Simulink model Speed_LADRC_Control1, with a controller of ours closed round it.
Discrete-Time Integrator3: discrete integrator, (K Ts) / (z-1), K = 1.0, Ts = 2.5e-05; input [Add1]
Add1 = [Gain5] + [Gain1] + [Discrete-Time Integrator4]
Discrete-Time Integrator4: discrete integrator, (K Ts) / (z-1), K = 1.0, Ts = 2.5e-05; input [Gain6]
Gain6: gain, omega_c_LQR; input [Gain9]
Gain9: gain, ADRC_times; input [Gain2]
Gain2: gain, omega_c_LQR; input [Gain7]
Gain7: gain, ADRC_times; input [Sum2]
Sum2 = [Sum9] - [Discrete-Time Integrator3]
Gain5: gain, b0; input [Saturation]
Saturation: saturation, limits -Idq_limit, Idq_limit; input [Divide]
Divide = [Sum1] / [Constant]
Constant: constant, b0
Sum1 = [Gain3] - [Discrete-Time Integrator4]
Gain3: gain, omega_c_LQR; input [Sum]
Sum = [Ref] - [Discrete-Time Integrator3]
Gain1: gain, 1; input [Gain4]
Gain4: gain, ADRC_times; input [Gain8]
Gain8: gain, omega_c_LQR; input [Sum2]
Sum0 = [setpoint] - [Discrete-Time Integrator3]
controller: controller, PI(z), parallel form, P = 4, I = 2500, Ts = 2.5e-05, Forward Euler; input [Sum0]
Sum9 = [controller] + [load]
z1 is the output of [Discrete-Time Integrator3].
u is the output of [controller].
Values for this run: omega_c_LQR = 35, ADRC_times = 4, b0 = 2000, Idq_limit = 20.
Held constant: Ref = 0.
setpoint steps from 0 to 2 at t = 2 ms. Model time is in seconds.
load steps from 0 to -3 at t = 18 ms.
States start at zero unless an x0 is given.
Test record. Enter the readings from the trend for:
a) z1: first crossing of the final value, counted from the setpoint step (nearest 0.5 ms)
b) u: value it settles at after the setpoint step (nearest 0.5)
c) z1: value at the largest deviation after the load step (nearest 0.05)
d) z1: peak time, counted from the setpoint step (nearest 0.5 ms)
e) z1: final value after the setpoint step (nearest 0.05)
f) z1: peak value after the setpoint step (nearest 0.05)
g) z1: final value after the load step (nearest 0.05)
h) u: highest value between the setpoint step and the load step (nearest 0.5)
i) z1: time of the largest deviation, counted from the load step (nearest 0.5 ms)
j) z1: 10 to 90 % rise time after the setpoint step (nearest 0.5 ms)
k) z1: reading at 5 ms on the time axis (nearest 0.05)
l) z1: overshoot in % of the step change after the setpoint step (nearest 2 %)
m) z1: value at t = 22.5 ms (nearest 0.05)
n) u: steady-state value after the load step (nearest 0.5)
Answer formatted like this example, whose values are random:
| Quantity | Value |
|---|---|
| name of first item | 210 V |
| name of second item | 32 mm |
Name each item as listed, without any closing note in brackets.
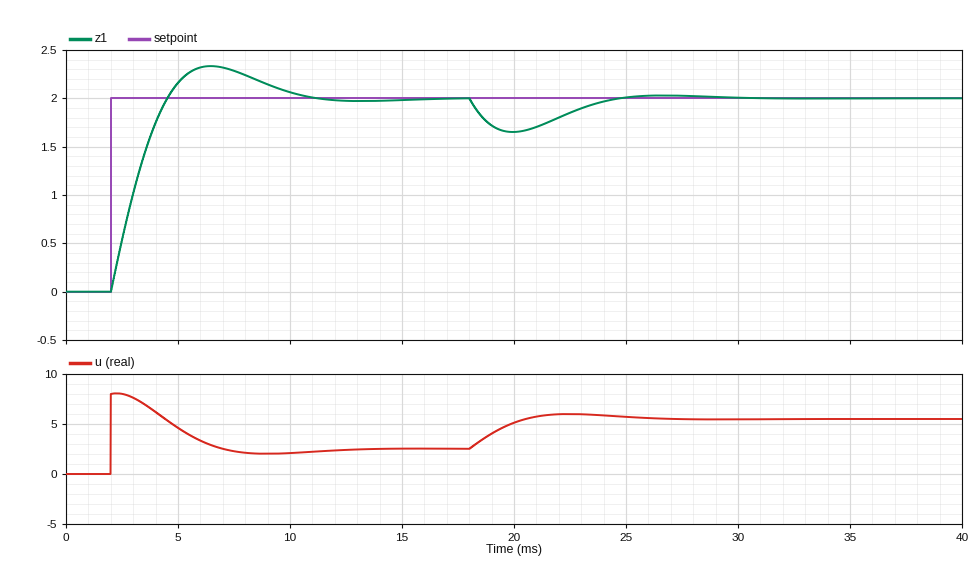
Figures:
| Quantity | Value |
|---|---|
| z1: first crossing of the final value, counted from the setpoint step | 2.5 ms |
| u: value it settles at after the setpoint step | 2.5 |
| z1: value at the largest deviation after the load step | 1.65 |
| z1: peak time, counted from the setpoint step | 4.5 ms |
| z1: final value after the setpoint step | 2.00 |
| z1: peak value after the setpoint step | 2.35 |
| z1: final value after the load step | 2.00 |
| u: highest value between the setpoint step and the load step | 8.0 |
| z1: time of the largest deviation, counted from the load step | 2.0 ms |
| z1: 10 to 90 % rise time after the setpoint step | 2.0 ms |
| z1: reading at 5 ms on the time axis | 2.15 |
| z1: overshoot in % of the step change after the setpoint step | 16 % |
| z1: value at t = 22.5 ms | 1.85 |
| u: steady-state value after the load step | 5.5 |
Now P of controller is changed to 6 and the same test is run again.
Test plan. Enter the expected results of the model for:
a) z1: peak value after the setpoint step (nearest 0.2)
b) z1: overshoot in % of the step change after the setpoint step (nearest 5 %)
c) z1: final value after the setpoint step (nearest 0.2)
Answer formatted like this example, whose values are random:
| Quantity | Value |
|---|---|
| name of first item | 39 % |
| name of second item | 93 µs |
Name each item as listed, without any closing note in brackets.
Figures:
| Quantity | Value |
|---|---|
| z1: peak value after the setpoint step | 2.2 |
| z1: overshoot in % of the step change after the setpoint step | 10 % |
| z1: final value after the setpoint step | 2.0 |
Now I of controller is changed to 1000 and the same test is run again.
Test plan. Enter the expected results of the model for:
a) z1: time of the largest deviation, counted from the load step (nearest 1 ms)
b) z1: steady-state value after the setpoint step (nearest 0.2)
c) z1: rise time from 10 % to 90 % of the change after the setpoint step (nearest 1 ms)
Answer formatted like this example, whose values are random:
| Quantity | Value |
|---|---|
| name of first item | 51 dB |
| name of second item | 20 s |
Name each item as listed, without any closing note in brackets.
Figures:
| Quantity | Value |
|---|---|
| z1: time of the largest deviation, counted from the load step | 3 ms |
| z1: steady-state value after the setpoint step | 2.0 |
| z1: rise time from 10 % to 90 % of the change after the setpoint step | 3 ms |
